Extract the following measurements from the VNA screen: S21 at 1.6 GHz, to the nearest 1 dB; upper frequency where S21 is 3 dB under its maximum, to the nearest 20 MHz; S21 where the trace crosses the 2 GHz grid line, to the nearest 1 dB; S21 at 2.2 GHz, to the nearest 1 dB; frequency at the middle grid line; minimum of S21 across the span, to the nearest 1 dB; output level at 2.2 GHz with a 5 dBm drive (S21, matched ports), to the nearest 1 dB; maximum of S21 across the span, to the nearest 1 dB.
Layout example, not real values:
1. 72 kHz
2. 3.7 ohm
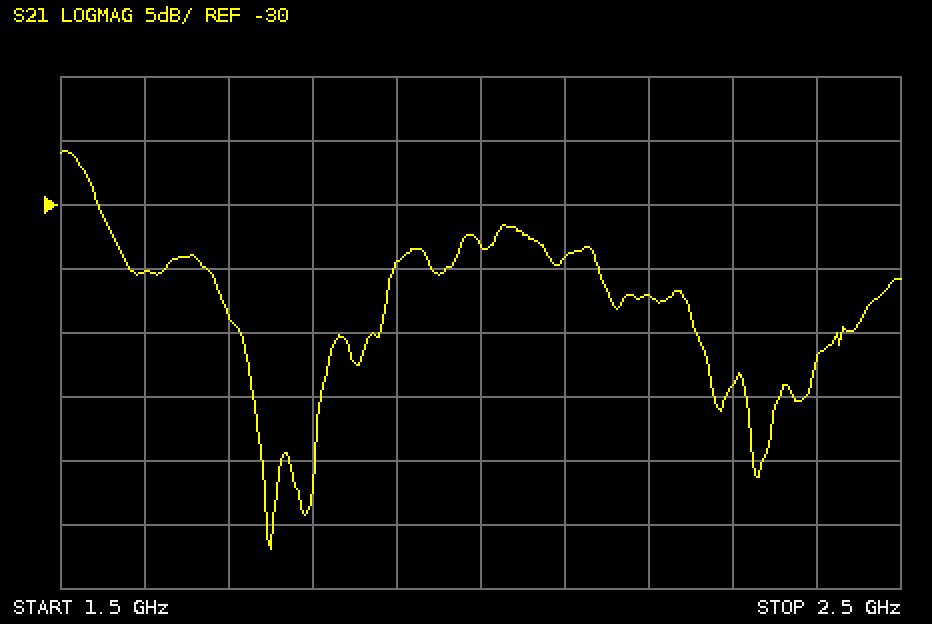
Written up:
1. -35 dB
2. 1.54 GHz
3. -33 dB
4. -37 dB
5. 2 GHz
6. -57 dB
7. -32 dBm
8. -26 dB
